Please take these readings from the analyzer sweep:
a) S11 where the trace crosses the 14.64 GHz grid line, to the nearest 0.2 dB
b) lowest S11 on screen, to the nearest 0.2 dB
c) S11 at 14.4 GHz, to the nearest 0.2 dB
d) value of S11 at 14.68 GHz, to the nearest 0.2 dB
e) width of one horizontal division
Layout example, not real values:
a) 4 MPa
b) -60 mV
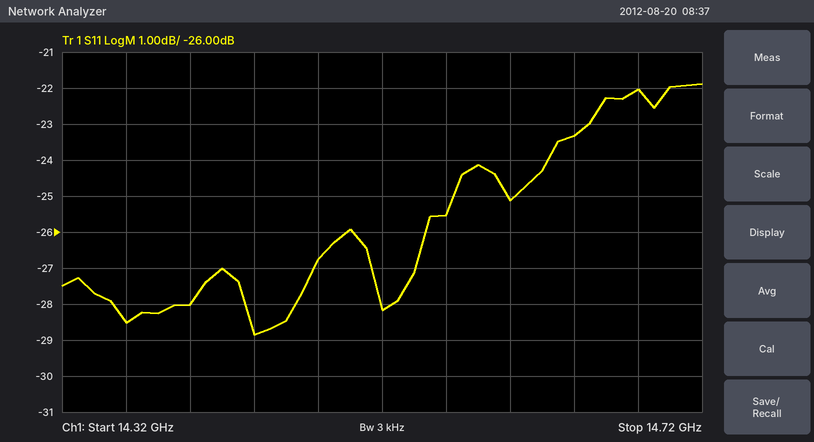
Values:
a) -23.4 dB
b) -28.8 dB
c) -28.0 dB
d) -22.0 dB
e) 40 MHz
